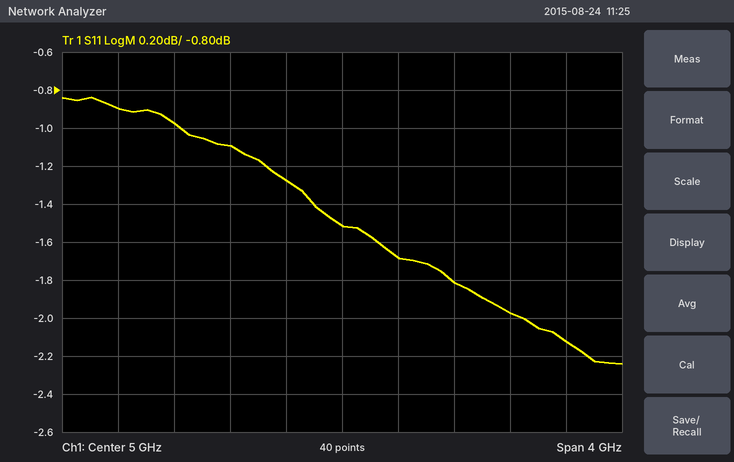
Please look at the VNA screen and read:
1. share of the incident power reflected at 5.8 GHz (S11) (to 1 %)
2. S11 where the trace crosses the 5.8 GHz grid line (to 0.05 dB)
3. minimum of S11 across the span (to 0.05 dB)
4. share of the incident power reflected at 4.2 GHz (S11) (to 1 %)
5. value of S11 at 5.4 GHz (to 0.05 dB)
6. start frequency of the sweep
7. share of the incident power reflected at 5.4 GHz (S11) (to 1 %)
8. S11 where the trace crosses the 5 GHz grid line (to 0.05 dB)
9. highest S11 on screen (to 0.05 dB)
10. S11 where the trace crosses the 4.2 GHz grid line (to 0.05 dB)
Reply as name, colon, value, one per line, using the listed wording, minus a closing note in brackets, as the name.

share of the incident power reflected at 5.8 GHz (S11): 66 %
S11 where the trace crosses the 5.8 GHz grid line: -1.80 dB
minimum of S11 across the span: -2.25 dB
share of the incident power reflected at 4.2 GHz (S11): 78 %
value of S11 at 5.4 GHz: -1.70 dB
start frequency of the sweep: 3 GHz
share of the incident power reflected at 5.4 GHz (S11): 68 %
S11 where the trace crosses the 5 GHz grid line: -1.50 dB
highest S11 on screen: -0.85 dB
S11 where the trace crosses the 4.2 GHz grid line: -1.10 dB
